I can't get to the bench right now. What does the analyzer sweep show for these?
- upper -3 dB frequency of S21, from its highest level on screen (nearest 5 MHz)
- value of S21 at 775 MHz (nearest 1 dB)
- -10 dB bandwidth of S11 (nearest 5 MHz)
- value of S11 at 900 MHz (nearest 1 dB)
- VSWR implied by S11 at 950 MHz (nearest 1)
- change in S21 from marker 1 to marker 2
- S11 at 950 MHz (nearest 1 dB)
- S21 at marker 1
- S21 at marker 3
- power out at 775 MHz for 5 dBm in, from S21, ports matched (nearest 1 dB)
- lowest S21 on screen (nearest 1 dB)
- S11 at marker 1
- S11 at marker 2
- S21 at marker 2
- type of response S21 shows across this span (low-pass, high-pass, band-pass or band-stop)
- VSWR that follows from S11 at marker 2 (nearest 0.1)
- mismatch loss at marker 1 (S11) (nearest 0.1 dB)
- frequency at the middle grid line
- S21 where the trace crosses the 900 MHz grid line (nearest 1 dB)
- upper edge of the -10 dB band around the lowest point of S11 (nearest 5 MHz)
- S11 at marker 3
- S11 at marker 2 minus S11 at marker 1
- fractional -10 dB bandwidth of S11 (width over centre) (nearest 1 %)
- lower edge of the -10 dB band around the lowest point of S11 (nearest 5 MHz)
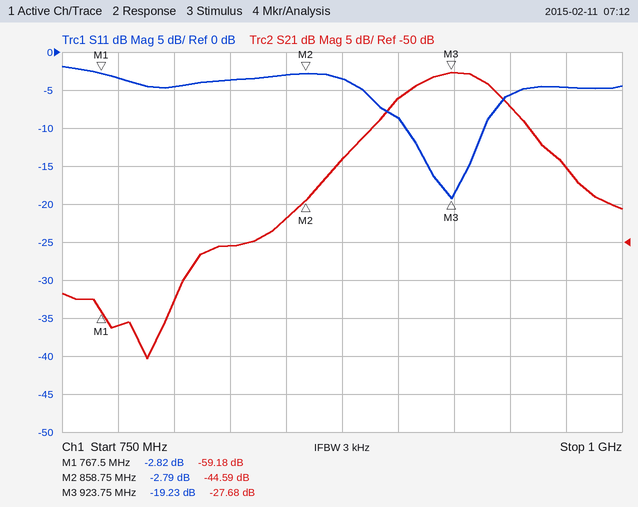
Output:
945 MHz
-61 dB
35 MHz
-9 dB
3
14.59 dB
-6 dB
-59.18 dB
-27.68 dB
-56 dBm
-65 dB
-2.82 dB
-2.79 dB
-44.59 dB
band-pass
6.3
3.2 dB
875 MHz
-31 dB
940 MHz
-19.23 dB
0.03 dB
4 %
905 MHz
